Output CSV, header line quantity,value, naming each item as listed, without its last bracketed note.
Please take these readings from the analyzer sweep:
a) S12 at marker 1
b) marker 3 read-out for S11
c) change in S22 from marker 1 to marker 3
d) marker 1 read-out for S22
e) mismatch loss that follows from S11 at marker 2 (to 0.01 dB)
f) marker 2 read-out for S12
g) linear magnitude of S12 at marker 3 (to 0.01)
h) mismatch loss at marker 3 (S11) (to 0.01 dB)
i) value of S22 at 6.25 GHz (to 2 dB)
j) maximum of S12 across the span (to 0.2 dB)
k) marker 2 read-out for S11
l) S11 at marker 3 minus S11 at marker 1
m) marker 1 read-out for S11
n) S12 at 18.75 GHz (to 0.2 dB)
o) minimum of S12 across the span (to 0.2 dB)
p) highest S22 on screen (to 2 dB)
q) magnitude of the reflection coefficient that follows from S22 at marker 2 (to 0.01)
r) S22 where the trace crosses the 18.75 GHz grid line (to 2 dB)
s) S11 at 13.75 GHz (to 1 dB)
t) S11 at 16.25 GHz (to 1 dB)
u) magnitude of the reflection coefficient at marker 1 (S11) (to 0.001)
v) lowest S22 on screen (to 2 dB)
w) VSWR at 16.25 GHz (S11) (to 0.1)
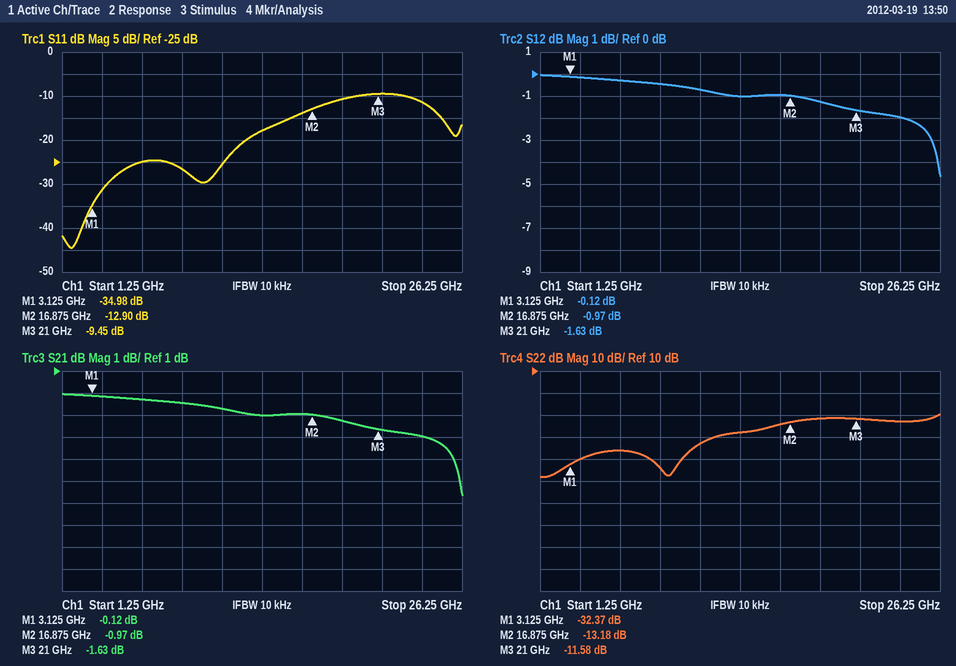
quantity,value
S12 at marker 1,-0.12 dB
marker 3 read-out for S11,-9.45 dB
change in S22 from marker 1 to marker 3,20.79 dB
marker 1 read-out for S22,-32.37 dB
mismatch loss that follows from S11 at marker 2,0.23 dB
marker 2 read-out for S12,-0.97 dB
linear magnitude of S12 at marker 3,0.83
mismatch loss at marker 3 (S11),0.52 dB
value of S22 at 6.25 GHz,-26 dB
maximum of S12 across the span,0.0 dB
marker 2 read-out for S11,-12.90 dB
S11 at marker 3 minus S11 at marker 1,25.53 dB
marker 1 read-out for S11,-34.98 dB
S12 at 18.75 GHz,-1.2 dB
minimum of S12 across the span,-4.6 dB
highest S22 on screen,-10 dB
magnitude of the reflection coefficient that follows from S22 at marker 2,0.22
S22 where the trace crosses the 18.75 GHz grid line,-12 dB
S11 at 13.75 GHz,-18 dB
S11 at 16.25 GHz,-14 dB
magnitude of the reflection coefficient at marker 1 (S11),0.018
lowest S22 on screen,-38 dB
VSWR at 16.25 GHz (S11),1.5
